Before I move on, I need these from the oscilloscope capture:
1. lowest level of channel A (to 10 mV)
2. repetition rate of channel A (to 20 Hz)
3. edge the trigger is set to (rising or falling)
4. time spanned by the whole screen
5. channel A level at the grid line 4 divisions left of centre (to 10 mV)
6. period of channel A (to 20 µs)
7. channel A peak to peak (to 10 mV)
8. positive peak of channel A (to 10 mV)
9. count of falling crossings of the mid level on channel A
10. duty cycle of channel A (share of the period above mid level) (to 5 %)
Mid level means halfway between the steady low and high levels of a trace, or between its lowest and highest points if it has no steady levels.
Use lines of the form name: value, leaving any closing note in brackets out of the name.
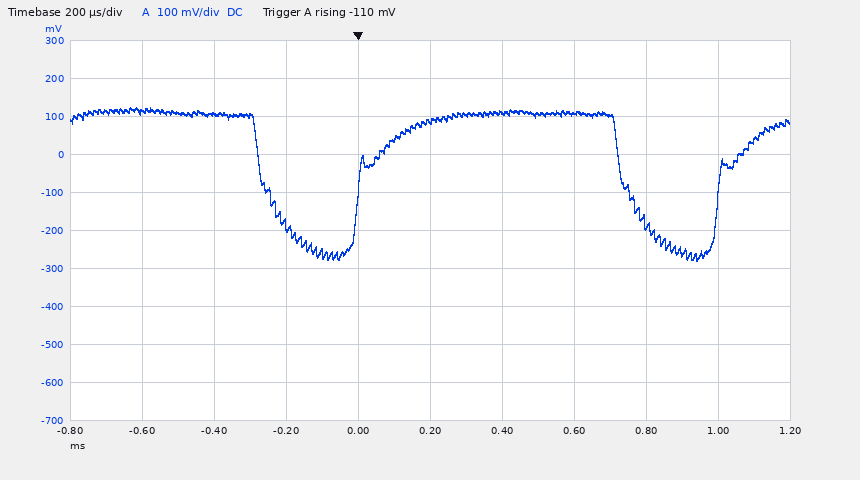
lowest level of channel A: -280 mV
repetition rate of channel A: 1.00 kHz
edge the trigger is set to: rising
time spanned by the whole screen: 2 ms
channel A level at the grid line 4 divisions left of centre: 110 mV
period of channel A: 1.00 ms
channel A peak to peak: 400 mV
positive peak of channel A: 120 mV
count of falling crossings of the mid level on channel A: 2
duty cycle of channel A (share of the period above mid level): 75 %
